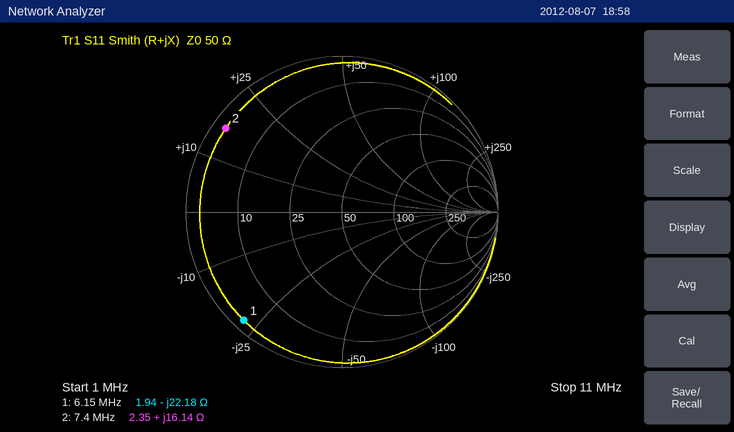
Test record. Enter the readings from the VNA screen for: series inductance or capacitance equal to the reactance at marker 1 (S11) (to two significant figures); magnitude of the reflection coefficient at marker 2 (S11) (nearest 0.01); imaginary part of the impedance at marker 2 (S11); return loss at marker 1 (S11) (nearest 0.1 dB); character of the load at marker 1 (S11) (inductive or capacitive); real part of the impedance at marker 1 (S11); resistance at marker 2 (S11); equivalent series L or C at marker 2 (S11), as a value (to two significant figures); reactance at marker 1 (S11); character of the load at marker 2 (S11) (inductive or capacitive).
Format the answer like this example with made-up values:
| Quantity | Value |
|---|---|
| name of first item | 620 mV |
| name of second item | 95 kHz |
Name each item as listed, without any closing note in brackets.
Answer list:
| Quantity | Value |
|---|---|
| series inductance or capacitance equal to the reactance at marker 1 (S11) | 1.2 nF |
| magnitude of the reflection coefficient at marker 2 (S11) | 0.92 |
| imaginary part of the impedance at marker 2 | +16.14 Ω |
| return loss at marker 1 (S11) | 0.6 dB |
| character of the load at marker 1 (S11) | capacitive |
| real part of the impedance at marker 1 | 1.94 Ω |
| resistance at marker 2 | 2.35 Ω |
| equivalent series L or C at marker 2 (S11), as a value | 350 nH |
| reactance at marker 1 | -22.18 Ω |
| character of the load at marker 2 (S11) | inductive |
